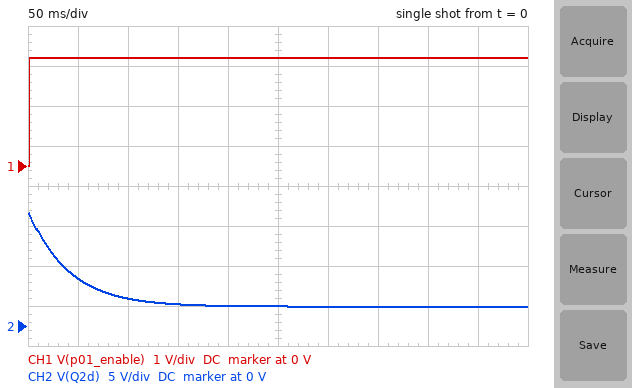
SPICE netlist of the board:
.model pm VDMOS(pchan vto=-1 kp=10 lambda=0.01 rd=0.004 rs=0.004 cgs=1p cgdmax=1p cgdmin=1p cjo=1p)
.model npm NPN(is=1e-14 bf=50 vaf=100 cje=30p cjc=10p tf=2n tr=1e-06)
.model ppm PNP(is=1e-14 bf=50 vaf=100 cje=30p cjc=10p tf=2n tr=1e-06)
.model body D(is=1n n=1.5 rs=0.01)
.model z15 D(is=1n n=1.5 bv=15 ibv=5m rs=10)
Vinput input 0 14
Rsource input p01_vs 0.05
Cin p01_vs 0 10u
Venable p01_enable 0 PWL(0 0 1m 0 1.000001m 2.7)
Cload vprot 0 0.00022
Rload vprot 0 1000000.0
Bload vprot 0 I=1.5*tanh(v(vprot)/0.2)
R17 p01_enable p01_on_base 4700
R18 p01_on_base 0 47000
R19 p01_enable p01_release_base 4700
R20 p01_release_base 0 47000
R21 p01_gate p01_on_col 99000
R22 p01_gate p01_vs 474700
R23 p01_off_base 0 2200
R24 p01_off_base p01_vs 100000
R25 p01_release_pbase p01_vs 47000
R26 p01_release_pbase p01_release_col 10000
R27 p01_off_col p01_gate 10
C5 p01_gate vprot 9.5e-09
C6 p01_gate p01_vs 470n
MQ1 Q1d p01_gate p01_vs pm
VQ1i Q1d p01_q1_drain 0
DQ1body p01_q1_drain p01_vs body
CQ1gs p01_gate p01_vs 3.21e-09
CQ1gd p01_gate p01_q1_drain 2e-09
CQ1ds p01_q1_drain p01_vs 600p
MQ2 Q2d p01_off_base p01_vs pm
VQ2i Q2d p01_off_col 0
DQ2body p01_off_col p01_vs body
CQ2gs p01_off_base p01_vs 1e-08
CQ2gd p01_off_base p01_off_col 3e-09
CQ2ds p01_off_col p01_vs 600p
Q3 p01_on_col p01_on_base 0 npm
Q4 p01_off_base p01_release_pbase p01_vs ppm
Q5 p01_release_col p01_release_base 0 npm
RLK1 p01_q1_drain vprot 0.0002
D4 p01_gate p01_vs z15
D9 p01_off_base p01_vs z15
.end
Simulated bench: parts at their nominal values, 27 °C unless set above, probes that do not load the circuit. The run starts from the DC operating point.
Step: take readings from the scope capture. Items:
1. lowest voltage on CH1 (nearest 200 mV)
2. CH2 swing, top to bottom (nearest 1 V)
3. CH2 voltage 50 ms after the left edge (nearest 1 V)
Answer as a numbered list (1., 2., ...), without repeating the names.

1. 0 V
2. 12 V
3. 6 V
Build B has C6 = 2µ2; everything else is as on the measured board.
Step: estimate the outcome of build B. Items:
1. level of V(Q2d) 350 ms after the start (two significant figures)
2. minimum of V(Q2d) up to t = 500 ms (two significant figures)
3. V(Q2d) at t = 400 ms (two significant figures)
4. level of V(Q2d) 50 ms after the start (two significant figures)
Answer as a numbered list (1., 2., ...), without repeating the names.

1. 4.1 V
2. 3.2 V
3. 3.7 V
4. 11 V
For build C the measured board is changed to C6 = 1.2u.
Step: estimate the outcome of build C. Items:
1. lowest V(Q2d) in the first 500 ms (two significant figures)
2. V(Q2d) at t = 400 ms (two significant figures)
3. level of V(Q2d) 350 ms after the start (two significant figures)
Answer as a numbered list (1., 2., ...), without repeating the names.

1. 2.5 V
2. 2.6 V
3. 2.8 V
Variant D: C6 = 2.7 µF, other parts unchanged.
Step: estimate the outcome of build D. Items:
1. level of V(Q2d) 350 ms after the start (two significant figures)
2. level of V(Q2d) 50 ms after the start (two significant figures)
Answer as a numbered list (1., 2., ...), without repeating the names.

1. 4.8 V
2. 12 V
